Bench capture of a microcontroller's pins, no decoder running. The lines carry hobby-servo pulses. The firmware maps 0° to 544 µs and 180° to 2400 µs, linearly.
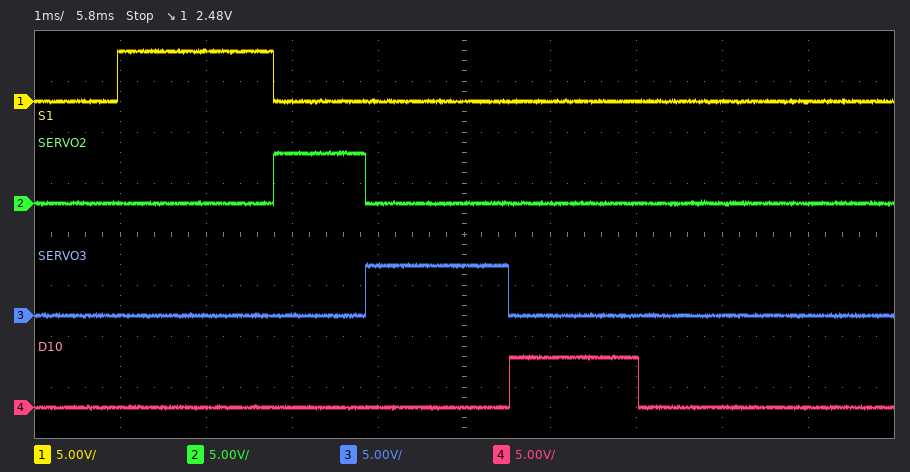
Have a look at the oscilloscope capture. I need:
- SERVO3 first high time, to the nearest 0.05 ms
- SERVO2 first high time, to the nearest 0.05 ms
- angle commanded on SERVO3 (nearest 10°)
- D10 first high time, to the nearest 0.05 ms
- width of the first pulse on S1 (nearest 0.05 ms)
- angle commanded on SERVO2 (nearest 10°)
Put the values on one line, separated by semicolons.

1.65 ms; 1.05 ms; 110°; 1.50 ms; 1.80 ms; 50°
